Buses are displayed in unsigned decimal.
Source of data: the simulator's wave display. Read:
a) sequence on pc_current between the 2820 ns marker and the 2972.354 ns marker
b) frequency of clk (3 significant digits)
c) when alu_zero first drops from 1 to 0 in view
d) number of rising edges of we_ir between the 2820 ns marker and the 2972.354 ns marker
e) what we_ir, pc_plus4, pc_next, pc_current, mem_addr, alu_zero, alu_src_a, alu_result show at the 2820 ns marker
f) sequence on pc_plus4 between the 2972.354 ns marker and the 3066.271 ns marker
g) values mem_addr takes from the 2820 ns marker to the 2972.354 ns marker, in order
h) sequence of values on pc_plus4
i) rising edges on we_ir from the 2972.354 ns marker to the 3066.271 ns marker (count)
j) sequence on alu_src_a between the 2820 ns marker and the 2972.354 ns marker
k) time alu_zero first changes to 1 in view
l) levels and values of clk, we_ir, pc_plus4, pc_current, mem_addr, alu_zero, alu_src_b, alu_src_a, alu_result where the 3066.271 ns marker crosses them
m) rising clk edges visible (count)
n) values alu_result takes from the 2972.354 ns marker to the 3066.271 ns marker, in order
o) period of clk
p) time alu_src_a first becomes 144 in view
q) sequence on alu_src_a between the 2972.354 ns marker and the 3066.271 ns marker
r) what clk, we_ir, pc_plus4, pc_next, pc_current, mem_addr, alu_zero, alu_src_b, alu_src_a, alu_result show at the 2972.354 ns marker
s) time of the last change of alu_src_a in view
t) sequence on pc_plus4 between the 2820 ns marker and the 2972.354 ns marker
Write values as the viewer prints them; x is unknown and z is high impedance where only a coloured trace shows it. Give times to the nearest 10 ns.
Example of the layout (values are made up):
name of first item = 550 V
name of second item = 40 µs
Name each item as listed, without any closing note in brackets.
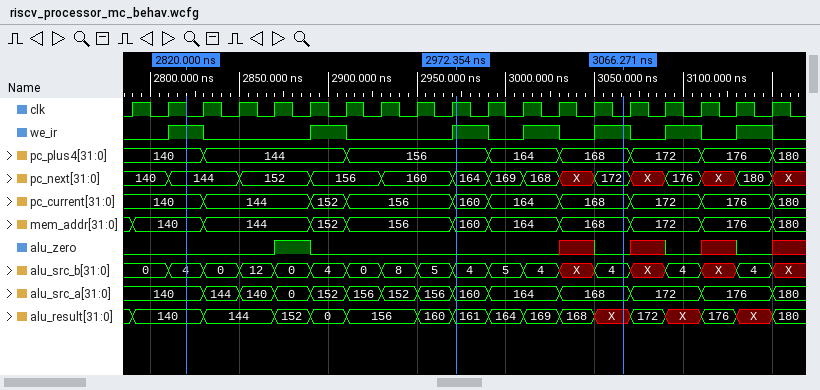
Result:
sequence on pc_current between the 2820 ns marker and the 2972.354 ns marker = 140, 144, 152, 156, 160
frequency of clk = 50.0 MHz
when alu_zero first drops from 1 to 0 in view = 2890 ns
number of rising edges of we_ir between the 2820 ns marker and the 2972.354 ns marker = 2
what we_ir, pc_plus4, pc_next, pc_current, mem_addr, alu_zero, alu_src_a, alu_result show at the 2820 ns marker = we_ir=1, pc_plus4=140, pc_next=144, pc_current=140, mem_addr=140, alu_zero=0, alu_src_a=140, alu_result=140
sequence on pc_plus4 between the 2972.354 ns marker and the 3066.271 ns marker = 156, 164, 168
values mem_addr takes from the 2820 ns marker to the 2972.354 ns marker, in order = 140, 144, 152, 156, 160
sequence of values on pc_plus4 = 140, 144, 156, 164, 168, 172, 176, 180
rising edges on we_ir from the 2972.354 ns marker to the 3066.271 ns marker = 2
sequence on alu_src_a between the 2820 ns marker and the 2972.354 ns marker = 140, 144, 140, 0, 152, 156, 152, 156, 160
time alu_zero first changes to 1 in view = 2870 ns
levels and values of clk, we_ir, pc_plus4, pc_current, mem_addr, alu_zero, alu_src_b, alu_src_a, alu_result where the 3066.271 ns marker crosses them = clk=0, we_ir=1, pc_plus4=168, pc_current=168, mem_addr=168, alu_zero=0, alu_src_b=4, alu_src_a=168, alu_result=X
rising clk edges visible = 19
values alu_result takes from the 2972.354 ns marker to the 3066.271 ns marker, in order = 161, 164, 169, 168, X
period of clk = 20 ns
time alu_src_a first becomes 144 in view = 2830 ns
sequence on alu_src_a between the 2972.354 ns marker and the 3066.271 ns marker = 160, 164, 168
what clk, we_ir, pc_plus4, pc_next, pc_current, mem_addr, alu_zero, alu_src_b, alu_src_a, alu_result show at the 2972.354 ns marker = clk=1, we_ir=1, pc_plus4=156, pc_next=164, pc_current=160, mem_addr=160, alu_zero=0, alu_src_b=4, alu_src_a=160, alu_result=161
time of the last change of alu_src_a in view = 3150 ns
sequence on pc_plus4 between the 2820 ns marker and the 2972.354 ns marker = 140, 144, 156
